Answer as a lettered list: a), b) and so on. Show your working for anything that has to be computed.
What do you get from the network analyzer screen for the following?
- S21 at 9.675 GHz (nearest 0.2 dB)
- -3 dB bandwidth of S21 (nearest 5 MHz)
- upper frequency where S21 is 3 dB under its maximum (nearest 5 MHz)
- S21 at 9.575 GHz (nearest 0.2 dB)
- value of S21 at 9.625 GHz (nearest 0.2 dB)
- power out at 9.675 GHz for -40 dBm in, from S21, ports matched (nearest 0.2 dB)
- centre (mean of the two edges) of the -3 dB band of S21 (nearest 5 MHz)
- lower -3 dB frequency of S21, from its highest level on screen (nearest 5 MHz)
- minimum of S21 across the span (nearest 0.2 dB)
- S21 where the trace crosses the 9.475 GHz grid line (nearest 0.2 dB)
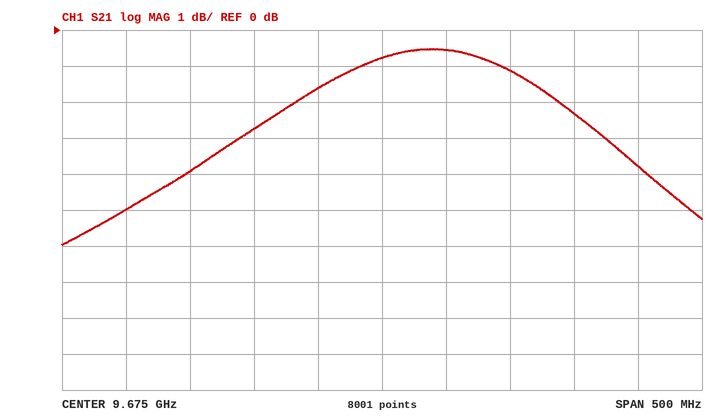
a) -0.8 dB
b) 9.865 GHz − 9.540 GHz = 325 MHz
c) 9.865 GHz
d) -2.8 dB
e) -1.6 dB
f) -40 dBm + (-0.8 dB) = -40.8 dBm
g) 9.705 GHz
h) 9.540 GHz
i) -6.0 dB
j) -5.0 dB
